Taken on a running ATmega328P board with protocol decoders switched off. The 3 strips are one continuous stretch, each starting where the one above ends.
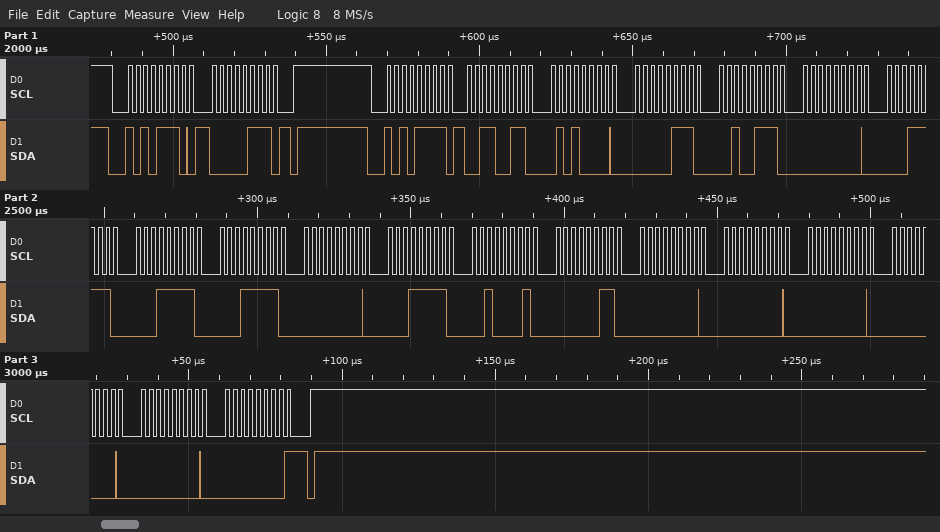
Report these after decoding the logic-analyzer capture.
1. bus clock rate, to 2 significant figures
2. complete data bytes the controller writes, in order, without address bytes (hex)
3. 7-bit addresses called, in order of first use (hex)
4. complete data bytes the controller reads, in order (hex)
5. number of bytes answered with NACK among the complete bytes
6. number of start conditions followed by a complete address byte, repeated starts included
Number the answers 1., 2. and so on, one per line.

1. 400 kHz
2. 07
3. 0x57
4. 33 50 07 27 00 1F 1F 1F 00 1F 21 03 00 00 00 00 00 00
5. 1
6. 2
